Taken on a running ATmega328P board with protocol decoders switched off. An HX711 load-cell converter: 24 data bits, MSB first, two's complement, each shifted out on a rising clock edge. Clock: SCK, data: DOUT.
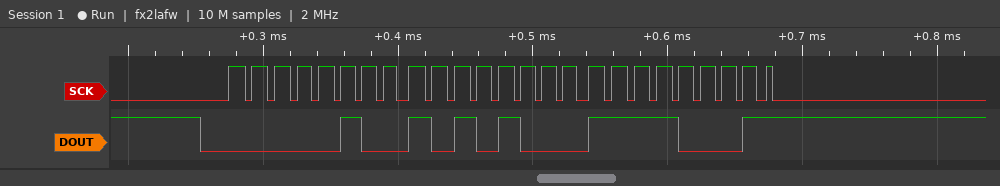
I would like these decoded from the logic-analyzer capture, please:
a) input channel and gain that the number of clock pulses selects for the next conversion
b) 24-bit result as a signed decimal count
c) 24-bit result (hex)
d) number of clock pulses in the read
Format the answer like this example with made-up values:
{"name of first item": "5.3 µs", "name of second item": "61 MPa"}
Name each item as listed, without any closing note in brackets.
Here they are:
{"input channel and gain that the number of clock pulses selects for the next conversion": "channel A, gain 128", "24-bit result as a signed decimal count": "305393", "24-bit result": "0x04A8F1", "number of clock pulses in the read": "25"}
